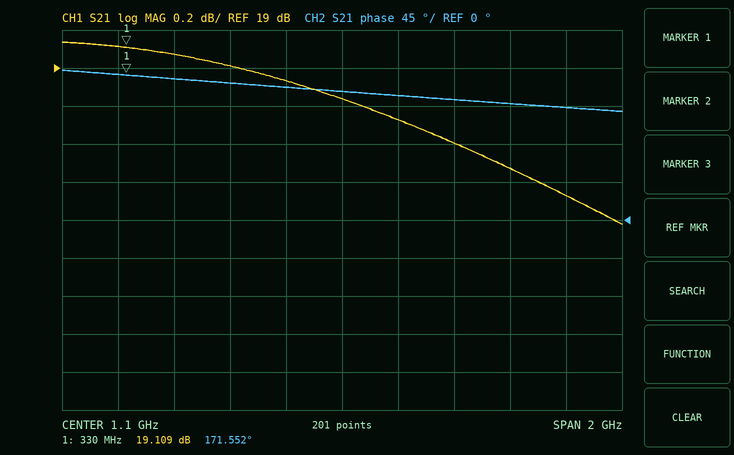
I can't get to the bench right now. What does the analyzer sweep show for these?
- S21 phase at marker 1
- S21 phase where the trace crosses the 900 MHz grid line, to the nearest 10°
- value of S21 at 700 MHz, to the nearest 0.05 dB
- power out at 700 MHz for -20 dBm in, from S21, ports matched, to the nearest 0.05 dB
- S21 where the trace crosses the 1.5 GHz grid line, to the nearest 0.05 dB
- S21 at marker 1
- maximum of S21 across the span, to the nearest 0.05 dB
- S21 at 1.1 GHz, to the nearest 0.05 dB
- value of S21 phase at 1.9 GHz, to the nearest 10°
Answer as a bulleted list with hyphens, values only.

- 171.552°
- 160°
- 19.00 dB
- -1.00 dBm
- 18.60 dB
- 19.109 dB
- 19.15 dB
- 18.85 dB
- 130°
